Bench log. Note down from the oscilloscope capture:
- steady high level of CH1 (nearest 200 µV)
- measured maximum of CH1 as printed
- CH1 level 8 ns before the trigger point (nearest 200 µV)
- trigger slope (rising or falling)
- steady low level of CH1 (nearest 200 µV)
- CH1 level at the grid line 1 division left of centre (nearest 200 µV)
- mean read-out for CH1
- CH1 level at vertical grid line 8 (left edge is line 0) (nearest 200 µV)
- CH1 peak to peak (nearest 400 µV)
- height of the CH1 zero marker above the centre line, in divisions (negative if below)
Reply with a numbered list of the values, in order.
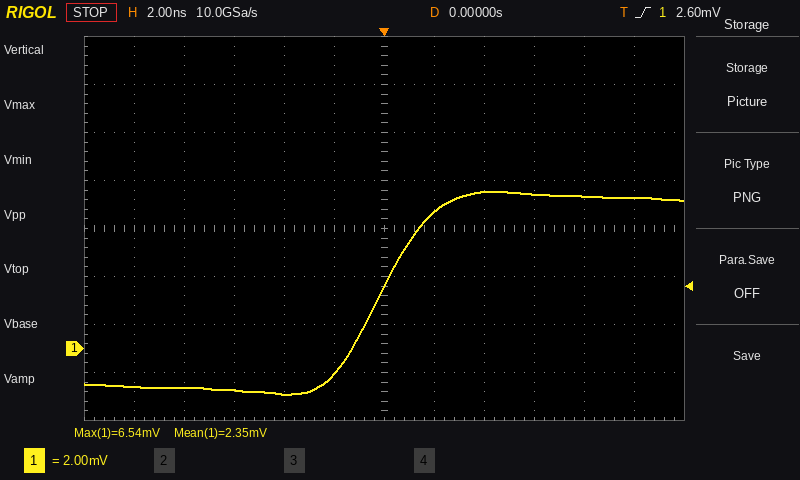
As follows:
1. 6.4 mV
2. 6.54 mV
3. -1.6 mV
4. rising
5. -1.6 mV
6. -1.0 mV
7. 2.35 mV
8. 6.6 mV
9. 8.4 mV
10. -2.5 div
